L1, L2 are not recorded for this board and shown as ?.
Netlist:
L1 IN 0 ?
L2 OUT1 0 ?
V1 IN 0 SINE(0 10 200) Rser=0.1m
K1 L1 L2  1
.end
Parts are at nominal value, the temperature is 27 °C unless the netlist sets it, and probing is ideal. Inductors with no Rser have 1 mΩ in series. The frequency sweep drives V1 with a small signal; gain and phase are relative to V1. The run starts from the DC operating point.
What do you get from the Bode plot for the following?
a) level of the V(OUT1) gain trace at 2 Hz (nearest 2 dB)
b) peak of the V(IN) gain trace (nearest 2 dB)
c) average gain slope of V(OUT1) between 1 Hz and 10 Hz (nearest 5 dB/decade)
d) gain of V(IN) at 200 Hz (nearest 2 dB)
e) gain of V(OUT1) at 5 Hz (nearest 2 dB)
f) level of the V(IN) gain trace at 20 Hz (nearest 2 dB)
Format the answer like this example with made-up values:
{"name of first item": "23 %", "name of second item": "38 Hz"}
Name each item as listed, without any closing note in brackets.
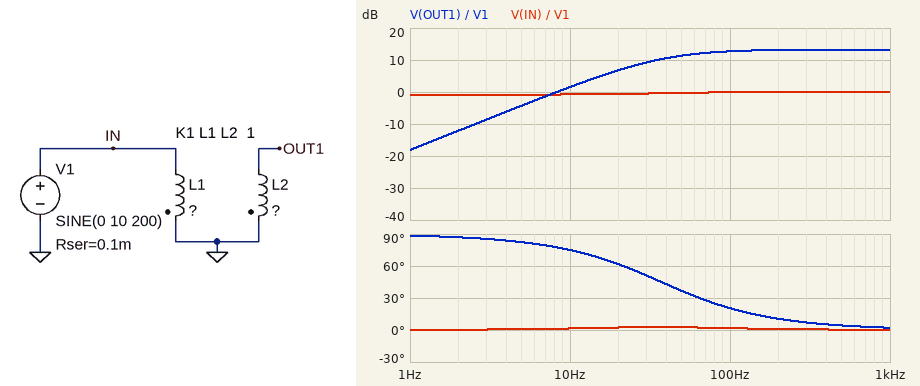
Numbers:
{"level of the V(OUT1) gain trace at 2 Hz": "-12 dB", "peak of the V(IN) gain trace": "0 dB", "average gain slope of V(OUT1) between 1 Hz and 10 Hz": "20 dB/decade", "gain of V(IN) at 200 Hz": "0 dB", "gain of V(OUT1) at 5 Hz": "-4 dB", "level of the V(IN) gain trace at 20 Hz": "0 dB"}
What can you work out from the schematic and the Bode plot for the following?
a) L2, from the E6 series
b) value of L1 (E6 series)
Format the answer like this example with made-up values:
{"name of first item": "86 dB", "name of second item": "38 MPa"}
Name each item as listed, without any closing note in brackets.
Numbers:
{"L2, from the E6 series": "100 µH", "value of L1": "4.7 µH"}
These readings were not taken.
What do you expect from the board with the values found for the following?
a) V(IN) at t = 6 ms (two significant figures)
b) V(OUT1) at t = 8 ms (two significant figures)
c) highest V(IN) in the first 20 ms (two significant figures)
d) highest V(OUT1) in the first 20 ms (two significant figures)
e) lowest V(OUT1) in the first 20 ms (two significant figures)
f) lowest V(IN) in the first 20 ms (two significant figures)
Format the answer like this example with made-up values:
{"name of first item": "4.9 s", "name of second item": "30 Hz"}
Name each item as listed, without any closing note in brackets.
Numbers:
{"V(IN) at t = 6 ms": "9.5 V", "V(OUT1) at t = 8 ms": "-34 V", "highest V(IN) in the first 20 ms": "10 V", "highest V(OUT1) in the first 20 ms": "45 V", "lowest V(OUT1) in the first 20 ms": "-49 V", "lowest V(IN) in the first 20 ms": "-10 V"}
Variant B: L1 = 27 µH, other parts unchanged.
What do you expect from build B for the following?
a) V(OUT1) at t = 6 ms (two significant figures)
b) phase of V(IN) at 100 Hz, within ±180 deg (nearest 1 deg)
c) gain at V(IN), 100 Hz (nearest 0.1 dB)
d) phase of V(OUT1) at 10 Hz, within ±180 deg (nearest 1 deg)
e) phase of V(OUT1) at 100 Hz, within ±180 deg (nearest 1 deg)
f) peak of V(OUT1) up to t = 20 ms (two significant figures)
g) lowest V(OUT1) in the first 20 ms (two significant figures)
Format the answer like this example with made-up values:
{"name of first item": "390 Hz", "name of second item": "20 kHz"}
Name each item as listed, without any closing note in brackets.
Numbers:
{"V(OUT1) at t = 6 ms": "18 V", "phase of V(IN) at 100 Hz, within ±180 deg": "0 deg", "gain at V(IN), 100 Hz": "0 dB", "phase of V(OUT1) at 10 Hz, within ±180 deg": "33 deg", "phase of V(OUT1) at 100 Hz, within ±180 deg": "4 deg", "peak of V(OUT1) up to t = 20 ms": "19 V", "lowest V(OUT1) in the first 20 ms": "-20 V"}
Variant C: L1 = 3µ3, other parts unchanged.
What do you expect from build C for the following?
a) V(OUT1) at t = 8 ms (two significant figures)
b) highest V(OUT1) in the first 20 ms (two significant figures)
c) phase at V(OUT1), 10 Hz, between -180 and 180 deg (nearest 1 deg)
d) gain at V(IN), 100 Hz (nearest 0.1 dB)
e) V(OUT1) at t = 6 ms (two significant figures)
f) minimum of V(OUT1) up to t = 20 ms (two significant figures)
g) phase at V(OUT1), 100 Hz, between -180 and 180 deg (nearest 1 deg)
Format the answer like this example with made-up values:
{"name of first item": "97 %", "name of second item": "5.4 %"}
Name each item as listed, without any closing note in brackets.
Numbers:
{"V(OUT1) at t = 8 ms": "-42 V", "highest V(OUT1) in the first 20 ms": "53 V", "phase at V(OUT1), 10 Hz, between -180 and 180 deg": "79 deg", "gain at V(IN), 100 Hz": "-0.2 dB", "V(OUT1) at t = 6 ms": "51 V", "minimum of V(OUT1) up to t = 20 ms": "-57 V", "phase at V(OUT1), 100 Hz, between -180 and 180 deg": "28 deg"}
